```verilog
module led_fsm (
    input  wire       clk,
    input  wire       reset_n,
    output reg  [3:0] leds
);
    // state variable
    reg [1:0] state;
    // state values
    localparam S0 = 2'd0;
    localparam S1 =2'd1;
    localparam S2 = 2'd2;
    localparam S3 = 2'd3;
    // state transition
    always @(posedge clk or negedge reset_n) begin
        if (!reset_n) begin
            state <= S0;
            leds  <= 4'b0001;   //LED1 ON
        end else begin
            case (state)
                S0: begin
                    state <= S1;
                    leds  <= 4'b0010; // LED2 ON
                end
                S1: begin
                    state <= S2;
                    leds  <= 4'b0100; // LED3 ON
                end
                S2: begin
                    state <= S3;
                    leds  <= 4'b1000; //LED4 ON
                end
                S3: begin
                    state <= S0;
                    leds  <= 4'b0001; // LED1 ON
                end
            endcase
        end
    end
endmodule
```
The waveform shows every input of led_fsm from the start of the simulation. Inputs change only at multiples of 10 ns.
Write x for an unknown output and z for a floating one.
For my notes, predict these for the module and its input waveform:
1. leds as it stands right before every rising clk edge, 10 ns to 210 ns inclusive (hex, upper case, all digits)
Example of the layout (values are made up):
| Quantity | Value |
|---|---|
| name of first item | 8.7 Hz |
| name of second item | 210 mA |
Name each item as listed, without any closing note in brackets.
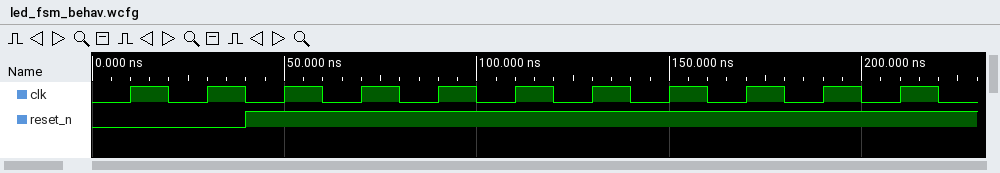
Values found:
| Quantity | Value |
|---|---|
| leds as it stands right before every rising clk edge, 10 ns to 210 ns inclusive | 1, 1, 1, 2, 4, 8, 1, 2, 4, 8, 1 |
